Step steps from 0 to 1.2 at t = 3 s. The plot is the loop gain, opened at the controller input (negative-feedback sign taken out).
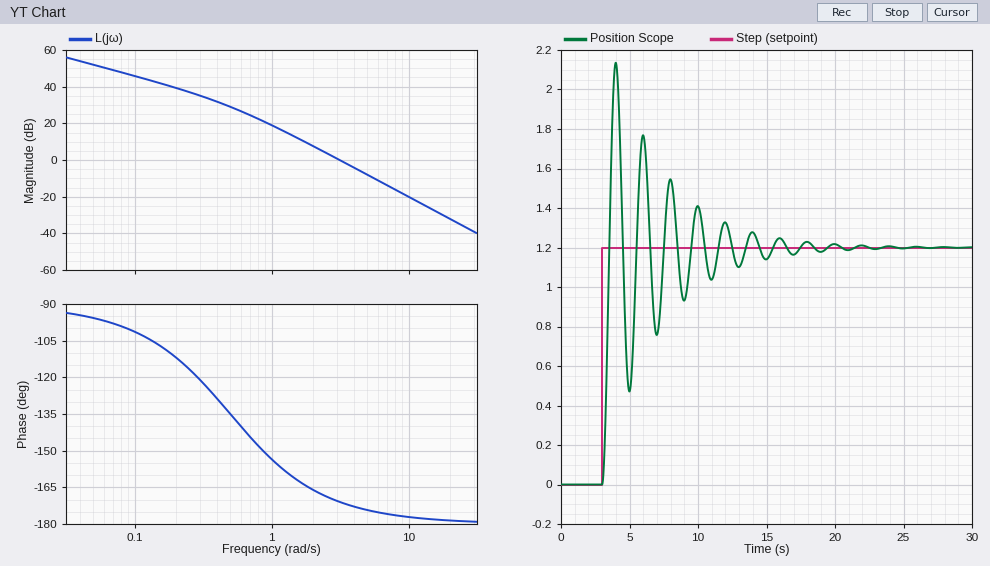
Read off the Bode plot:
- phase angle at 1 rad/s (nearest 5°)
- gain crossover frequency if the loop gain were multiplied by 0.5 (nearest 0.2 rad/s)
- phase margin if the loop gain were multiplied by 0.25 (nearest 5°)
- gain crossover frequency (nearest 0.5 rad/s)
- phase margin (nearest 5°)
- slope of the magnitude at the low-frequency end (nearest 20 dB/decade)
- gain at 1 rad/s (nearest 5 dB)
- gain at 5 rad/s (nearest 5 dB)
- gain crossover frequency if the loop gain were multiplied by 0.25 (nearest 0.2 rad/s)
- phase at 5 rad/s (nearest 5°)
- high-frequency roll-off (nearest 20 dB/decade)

-155°
2.2 rad/s
20°
3.0 rad/s
10°
-20 dB/decade
20 dB
-10 dB
1.6 rad/s
-175°
-40 dB/decade
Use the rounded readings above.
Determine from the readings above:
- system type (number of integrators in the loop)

1
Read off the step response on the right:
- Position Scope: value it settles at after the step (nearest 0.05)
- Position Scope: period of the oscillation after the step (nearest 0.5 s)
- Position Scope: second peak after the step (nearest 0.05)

1.20
2.0 s
1.75
